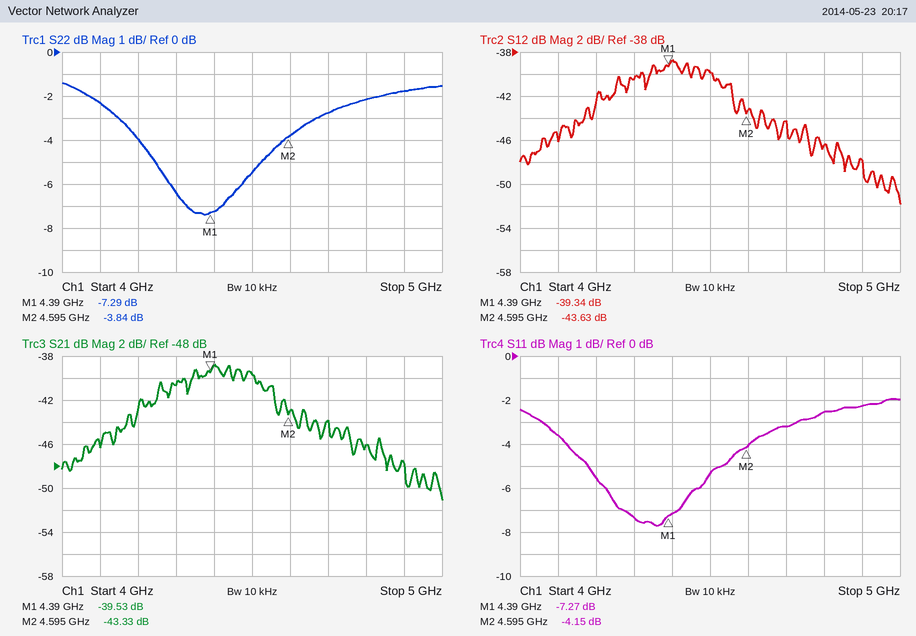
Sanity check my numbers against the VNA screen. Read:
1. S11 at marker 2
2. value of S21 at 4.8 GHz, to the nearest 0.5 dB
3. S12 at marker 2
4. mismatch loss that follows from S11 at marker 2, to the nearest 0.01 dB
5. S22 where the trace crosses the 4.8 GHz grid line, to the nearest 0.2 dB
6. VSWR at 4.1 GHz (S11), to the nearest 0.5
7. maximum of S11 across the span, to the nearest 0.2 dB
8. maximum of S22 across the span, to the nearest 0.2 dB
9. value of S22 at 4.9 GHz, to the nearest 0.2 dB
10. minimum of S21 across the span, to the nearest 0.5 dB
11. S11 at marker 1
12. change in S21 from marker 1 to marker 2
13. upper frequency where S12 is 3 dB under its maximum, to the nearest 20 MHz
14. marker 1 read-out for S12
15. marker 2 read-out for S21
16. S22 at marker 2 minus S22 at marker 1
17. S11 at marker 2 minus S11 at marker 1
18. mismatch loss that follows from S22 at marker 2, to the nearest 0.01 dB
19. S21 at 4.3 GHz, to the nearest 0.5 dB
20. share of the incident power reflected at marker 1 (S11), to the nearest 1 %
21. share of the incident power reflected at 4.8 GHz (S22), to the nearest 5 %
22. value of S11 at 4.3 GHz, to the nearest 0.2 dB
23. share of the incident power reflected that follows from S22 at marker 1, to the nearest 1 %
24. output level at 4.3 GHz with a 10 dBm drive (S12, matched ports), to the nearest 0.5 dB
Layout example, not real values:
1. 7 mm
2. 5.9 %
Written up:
1. -4.15 dB
2. -46.0 dB
3. -43.63 dB
4. 2.11 dB
5. -2.2 dB
6. 5.0
7. -2.0 dB
8. -1.4 dB
9. -1.8 dB
10. -51.0 dB
11. -7.27 dB
12. -3.80 dB
13. 4.56 GHz
14. -39.34 dB
15. -43.33 dB
16. 3.45 dB
17. 3.12 dB
18. 2.31 dB
19. -40.5 dB
20. 19 %
21. 60 %
22. -7.4 dB
23. 19 %
24. -30.5 dBm
